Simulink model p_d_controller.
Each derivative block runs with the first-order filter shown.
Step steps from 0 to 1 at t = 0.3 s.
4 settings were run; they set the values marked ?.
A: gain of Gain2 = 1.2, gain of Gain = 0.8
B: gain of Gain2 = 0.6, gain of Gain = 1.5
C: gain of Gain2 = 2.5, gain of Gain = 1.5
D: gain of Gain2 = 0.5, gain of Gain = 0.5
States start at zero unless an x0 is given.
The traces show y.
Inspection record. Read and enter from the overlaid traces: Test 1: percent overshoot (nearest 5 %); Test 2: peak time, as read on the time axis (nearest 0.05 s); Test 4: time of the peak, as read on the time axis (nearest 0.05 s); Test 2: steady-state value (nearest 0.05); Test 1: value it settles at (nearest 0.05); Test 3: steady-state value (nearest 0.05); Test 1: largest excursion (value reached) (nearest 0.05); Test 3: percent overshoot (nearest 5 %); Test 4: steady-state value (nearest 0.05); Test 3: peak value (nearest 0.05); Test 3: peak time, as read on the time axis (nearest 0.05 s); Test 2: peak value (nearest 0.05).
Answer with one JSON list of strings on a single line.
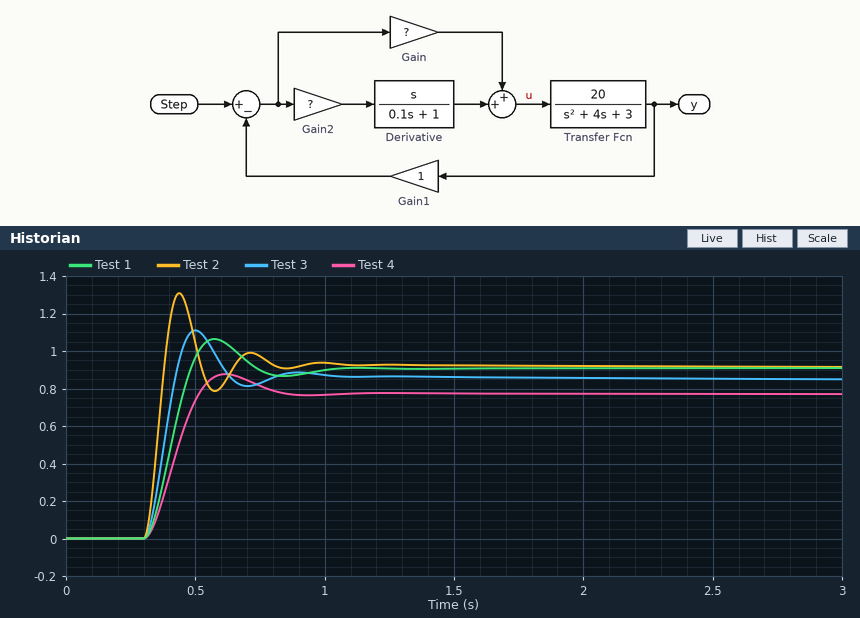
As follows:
["15 %", "0.45 s", "0.60 s", "0.90", "0.90", "0.85", "1.05", "30 %", "0.75", "1.10", "0.50 s", "1.30"]
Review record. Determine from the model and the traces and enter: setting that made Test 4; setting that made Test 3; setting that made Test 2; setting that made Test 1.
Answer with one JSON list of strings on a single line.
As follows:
["D", "A", "C", "B"]
